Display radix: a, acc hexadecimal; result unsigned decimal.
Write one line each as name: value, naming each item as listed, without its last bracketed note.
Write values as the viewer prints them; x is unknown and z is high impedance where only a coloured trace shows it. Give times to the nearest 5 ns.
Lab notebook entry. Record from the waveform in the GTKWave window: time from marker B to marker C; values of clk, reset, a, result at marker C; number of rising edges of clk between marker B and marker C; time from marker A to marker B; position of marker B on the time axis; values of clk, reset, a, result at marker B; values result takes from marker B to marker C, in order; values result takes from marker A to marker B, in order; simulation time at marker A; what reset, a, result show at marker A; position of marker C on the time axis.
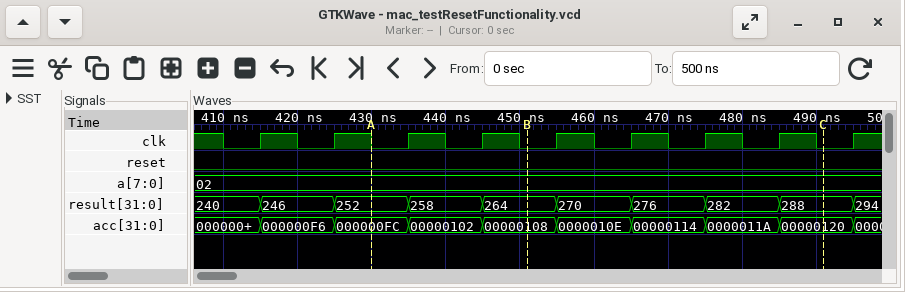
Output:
time from marker B to marker C: 40 ns
values of clk, reset, a, result at marker C: clk=0, reset=0, a=02, result=288
number of rising edges of clk between marker B and marker C: 4
time from marker A to marker B: 20 ns
position of marker B on the time axis: 450 ns
values of clk, reset, a, result at marker B: clk=0, reset=0, a=02, result=264
values result takes from marker B to marker C, in order: 264, 270, 276, 282, 288
values result takes from marker A to marker B, in order: 252, 258, 264
simulation time at marker A: 430 ns
what reset, a, result show at marker A: reset=0, a=02, result=252
position of marker C on the time axis: 490 ns
